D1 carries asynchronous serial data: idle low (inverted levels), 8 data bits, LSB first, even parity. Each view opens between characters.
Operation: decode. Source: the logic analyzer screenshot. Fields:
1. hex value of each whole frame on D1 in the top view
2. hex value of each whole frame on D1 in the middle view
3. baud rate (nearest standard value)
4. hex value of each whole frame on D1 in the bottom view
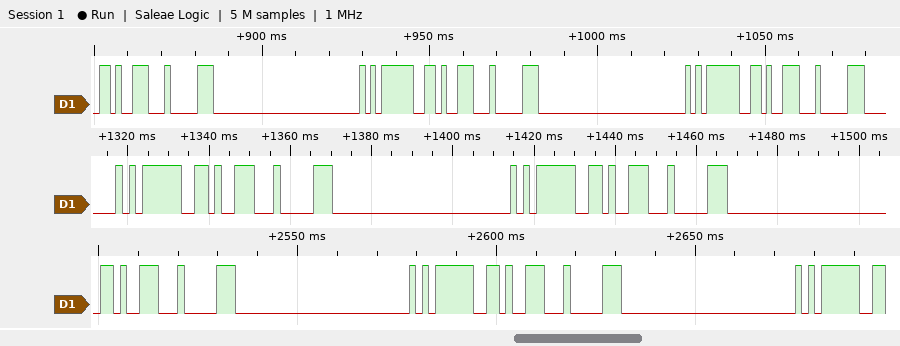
1A, 1F, 05, 1A, 1F, 05, 1A, 1F
05, 1A, 1F, 05, 1A, 1F
600 baud
1A, 1F, 05, 1A, 1F, 05
